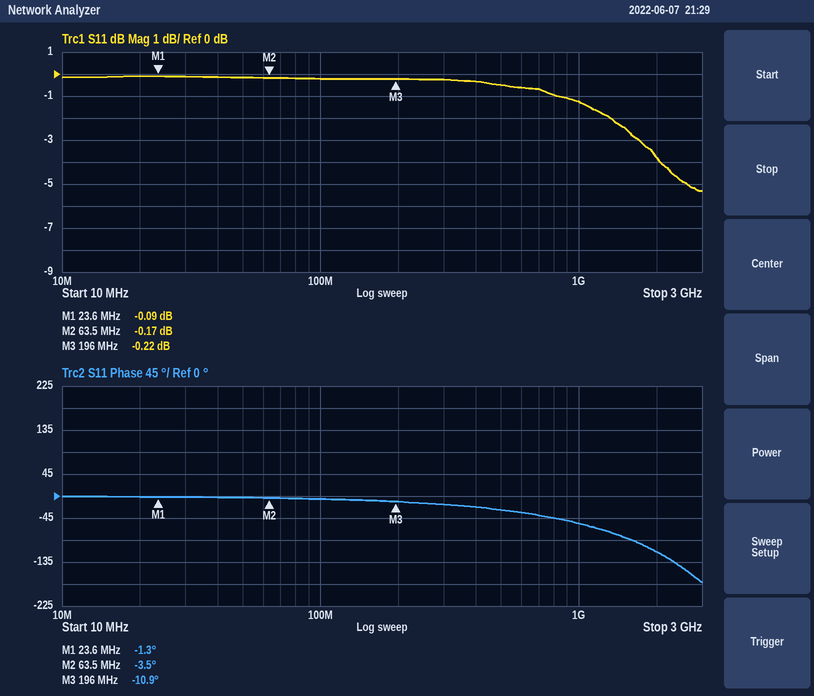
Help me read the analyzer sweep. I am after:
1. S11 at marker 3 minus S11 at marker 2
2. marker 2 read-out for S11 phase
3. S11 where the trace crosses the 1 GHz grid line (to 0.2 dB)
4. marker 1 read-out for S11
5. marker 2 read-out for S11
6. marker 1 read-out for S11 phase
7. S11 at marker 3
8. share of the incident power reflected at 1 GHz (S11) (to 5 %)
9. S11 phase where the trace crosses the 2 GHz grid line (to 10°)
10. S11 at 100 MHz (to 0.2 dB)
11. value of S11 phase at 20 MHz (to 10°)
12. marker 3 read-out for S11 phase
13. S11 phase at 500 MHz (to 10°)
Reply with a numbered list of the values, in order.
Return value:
1. -0.05 dB
2. -3.5°
3. -1.2 dB
4. -0.09 dB
5. -0.17 dB
6. -1.3°
7. -0.22 dB
8. 75 %
9. -110°
10. -0.2 dB
11. 0°
12. -10.9°
13. -30°
